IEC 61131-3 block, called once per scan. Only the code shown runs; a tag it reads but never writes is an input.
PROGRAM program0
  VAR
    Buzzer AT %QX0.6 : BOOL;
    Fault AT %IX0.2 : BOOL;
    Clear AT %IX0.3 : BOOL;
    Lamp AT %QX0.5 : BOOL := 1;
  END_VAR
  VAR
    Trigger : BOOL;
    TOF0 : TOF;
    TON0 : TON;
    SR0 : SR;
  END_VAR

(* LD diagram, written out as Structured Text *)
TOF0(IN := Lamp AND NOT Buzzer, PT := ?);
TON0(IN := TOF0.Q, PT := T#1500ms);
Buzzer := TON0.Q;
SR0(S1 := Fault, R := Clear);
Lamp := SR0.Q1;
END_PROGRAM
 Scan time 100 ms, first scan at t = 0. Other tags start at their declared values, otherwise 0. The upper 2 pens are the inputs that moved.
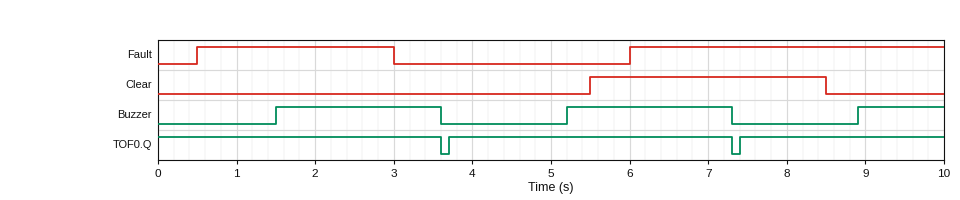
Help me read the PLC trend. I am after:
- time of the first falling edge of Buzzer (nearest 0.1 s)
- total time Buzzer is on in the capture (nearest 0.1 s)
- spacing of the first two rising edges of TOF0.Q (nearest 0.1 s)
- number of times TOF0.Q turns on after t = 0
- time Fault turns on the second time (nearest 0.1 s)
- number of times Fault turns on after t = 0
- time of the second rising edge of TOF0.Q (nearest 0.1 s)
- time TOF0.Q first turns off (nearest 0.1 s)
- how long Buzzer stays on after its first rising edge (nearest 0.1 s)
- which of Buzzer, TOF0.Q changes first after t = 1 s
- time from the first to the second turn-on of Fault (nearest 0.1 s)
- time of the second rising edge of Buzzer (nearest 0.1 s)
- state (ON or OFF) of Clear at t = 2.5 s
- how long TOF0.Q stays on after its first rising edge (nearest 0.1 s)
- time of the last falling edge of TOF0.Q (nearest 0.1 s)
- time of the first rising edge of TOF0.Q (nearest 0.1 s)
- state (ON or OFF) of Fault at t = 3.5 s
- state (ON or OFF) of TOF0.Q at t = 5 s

3.6 s
5.3 s
3.7 s
2
6.0 s
2
7.4 s
3.6 s
2.1 s
Buzzer
5.5 s
5.2 s
OFF
3.6 s
7.3 s
3.7 s
OFF
ON
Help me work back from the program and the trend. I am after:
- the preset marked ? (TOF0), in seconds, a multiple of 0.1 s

2.0 s
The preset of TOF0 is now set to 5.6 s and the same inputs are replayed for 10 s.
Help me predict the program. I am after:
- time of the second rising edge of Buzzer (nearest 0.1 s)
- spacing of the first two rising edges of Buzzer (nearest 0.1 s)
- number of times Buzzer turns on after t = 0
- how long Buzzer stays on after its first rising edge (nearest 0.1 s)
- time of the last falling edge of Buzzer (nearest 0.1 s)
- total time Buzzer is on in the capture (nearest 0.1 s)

8.8 s
7.3 s
2
5.7 s
7.2 s
6.9 s
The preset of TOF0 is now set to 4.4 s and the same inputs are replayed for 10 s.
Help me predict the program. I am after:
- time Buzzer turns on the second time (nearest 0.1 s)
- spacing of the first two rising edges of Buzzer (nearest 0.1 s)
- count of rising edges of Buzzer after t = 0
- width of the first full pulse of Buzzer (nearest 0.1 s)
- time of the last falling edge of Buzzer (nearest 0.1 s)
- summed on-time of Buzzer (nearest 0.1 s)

7.6 s
6.1 s
2
4.5 s
6.0 s
6.9 s
